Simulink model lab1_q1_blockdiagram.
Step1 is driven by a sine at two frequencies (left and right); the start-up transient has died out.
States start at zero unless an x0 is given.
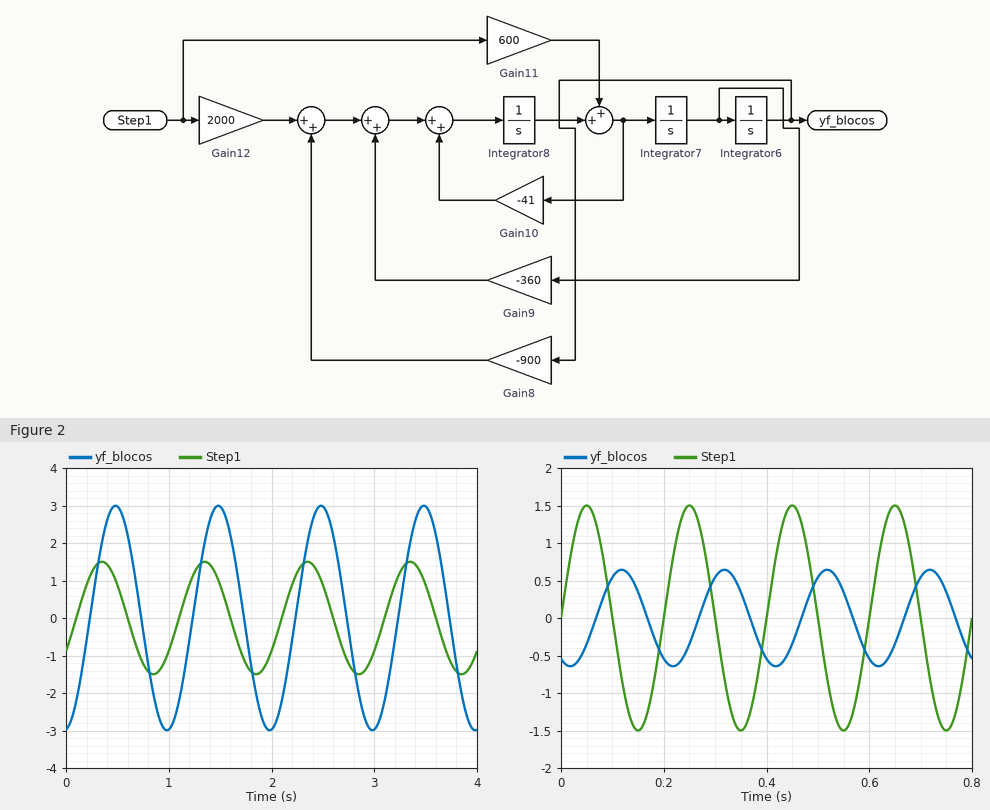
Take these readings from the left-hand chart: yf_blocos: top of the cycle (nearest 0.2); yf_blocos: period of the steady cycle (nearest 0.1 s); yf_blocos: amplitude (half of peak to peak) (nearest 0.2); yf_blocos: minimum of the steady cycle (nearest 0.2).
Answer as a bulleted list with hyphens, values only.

- 3.0
- 1.0 s
- 3.0
- -3.0
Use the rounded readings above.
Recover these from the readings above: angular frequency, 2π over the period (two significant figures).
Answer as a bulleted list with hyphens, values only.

- 6.3 rad/s
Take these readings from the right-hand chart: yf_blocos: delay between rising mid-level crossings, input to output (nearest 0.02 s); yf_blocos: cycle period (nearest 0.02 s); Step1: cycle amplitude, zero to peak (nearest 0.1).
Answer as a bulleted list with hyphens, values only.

- 0.06 s
- 0.20 s
- 1.5
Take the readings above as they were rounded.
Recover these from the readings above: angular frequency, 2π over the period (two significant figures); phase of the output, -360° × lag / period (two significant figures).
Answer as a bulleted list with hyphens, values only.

- 31 rad/s
- -110°
